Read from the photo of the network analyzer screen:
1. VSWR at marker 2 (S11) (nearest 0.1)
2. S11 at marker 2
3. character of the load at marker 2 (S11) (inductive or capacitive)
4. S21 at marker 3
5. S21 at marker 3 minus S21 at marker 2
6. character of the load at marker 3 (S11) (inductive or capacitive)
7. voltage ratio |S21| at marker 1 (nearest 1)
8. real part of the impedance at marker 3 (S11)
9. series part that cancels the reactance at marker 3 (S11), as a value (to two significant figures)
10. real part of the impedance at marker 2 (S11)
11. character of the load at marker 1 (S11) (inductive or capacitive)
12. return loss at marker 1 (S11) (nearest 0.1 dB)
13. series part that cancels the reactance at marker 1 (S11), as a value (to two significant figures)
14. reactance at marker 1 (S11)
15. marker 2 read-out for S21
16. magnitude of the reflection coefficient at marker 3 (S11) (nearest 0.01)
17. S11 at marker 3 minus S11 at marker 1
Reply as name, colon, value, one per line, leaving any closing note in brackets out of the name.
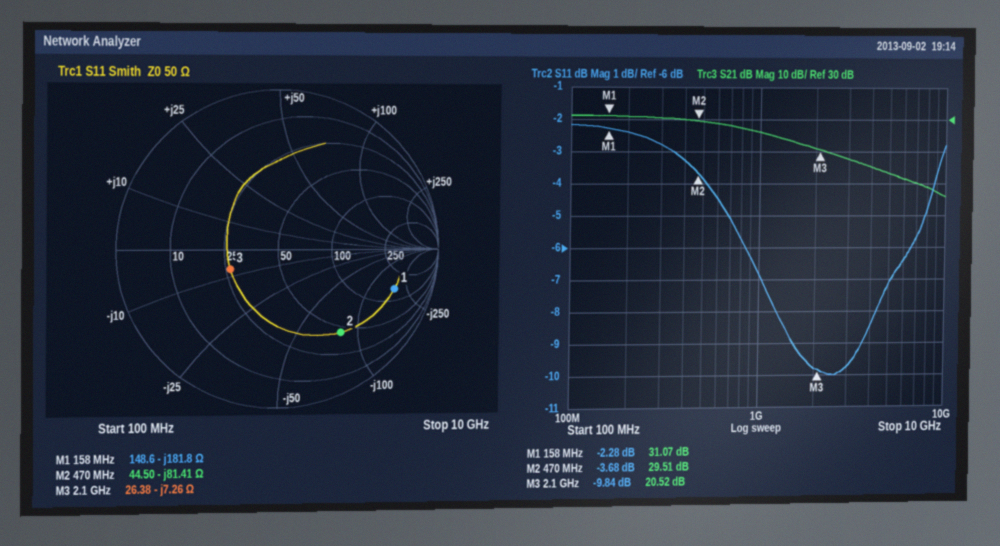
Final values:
VSWR at marker 2 (S11): 4.8
S11 at marker 2: -3.68 dB
character of the load at marker 2 (S11): capacitive
S21 at marker 3: 20.52 dB
S21 at marker 3 minus S21 at marker 2: -8.99 dB
character of the load at marker 3 (S11): capacitive
voltage ratio |S21| at marker 1: 36
real part of the impedance at marker 3: 26.38 Ω
series part that cancels the reactance at marker 3 (S11), as a value: 550 pH
real part of the impedance at marker 2: 44.50 Ω
character of the load at marker 1 (S11): capacitive
return loss at marker 1 (S11): 2.3 dB
series part that cancels the reactance at marker 1 (S11), as a value: 180 nH
reactance at marker 1: -181.8 Ω
marker 2 read-out for S21: 29.51 dB
magnitude of the reflection coefficient at marker 3 (S11): 0.32
S11 at marker 3 minus S11 at marker 1: -7.56 dB
